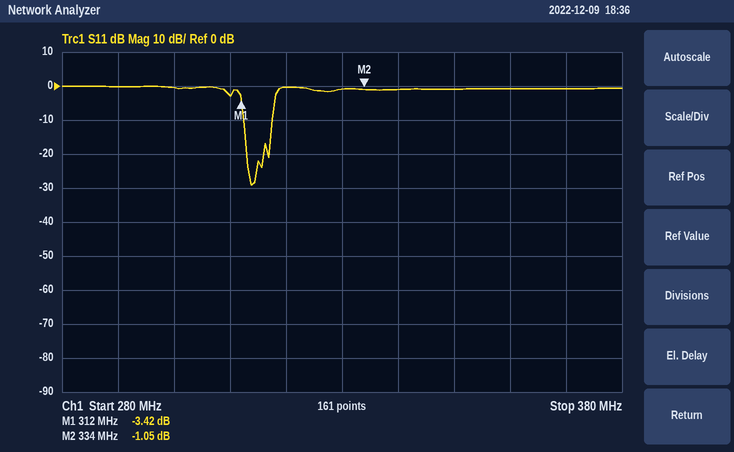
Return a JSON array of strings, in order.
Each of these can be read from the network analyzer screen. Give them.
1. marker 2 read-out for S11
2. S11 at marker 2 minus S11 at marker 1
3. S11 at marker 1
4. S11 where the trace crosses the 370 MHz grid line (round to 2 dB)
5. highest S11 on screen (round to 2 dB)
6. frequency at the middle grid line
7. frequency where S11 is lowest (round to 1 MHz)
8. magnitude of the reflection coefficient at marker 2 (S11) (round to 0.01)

["-1.05 dB", "2.37 dB", "-3.42 dB", "0 dB", "0 dB", "330 MHz", "314 MHz", "0.89"]
